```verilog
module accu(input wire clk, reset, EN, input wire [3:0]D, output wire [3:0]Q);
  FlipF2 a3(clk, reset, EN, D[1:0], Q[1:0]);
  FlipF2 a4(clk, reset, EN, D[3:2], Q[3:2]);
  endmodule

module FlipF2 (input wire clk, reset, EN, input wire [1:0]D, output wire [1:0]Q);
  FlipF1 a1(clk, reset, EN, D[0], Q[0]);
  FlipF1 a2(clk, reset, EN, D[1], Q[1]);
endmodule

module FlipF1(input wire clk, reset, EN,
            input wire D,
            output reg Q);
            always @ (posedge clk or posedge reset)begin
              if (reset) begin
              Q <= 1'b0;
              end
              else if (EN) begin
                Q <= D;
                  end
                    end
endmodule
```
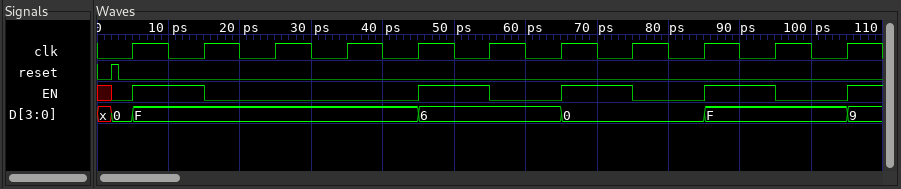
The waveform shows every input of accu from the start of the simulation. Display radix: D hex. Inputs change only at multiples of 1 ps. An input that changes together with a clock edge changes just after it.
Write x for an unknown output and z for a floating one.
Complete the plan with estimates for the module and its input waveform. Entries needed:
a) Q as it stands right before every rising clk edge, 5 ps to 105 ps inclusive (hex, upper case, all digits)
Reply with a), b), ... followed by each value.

a) 0, 0, F, F, F, F, 6, 6, 0, 0, F
